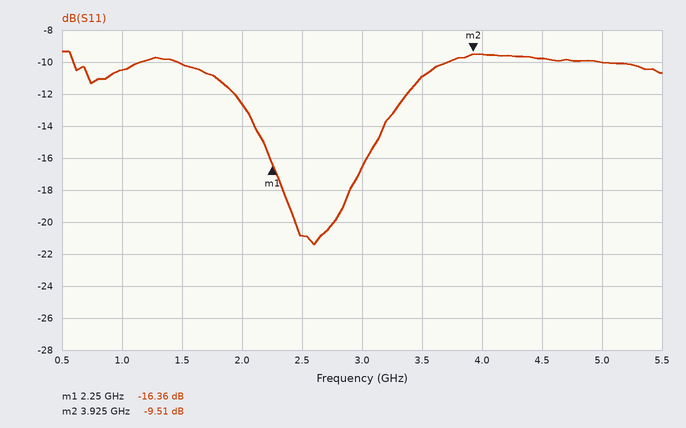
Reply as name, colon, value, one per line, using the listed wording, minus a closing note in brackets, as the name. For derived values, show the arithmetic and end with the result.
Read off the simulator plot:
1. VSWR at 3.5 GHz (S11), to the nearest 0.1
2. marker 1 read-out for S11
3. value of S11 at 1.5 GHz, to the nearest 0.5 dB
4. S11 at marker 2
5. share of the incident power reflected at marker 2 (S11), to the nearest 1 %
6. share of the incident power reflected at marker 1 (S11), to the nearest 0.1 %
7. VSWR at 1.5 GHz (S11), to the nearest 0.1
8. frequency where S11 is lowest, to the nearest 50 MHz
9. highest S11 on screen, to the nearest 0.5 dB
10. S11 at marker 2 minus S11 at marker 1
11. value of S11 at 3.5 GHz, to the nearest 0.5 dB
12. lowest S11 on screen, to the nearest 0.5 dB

VSWR at 3.5 GHz (S11), to the nearest 0.1: |Γ| = 10^(-11/20) = 0.2818; VSWR = (1 + 0.2818)/(1 − 0.2818) ≈ 1.8
marker 1 read-out for S11: -16.36 dB
value of S11 at 1.5 GHz, to the nearest 0.5 dB: -10.0 dB
S11 at marker 2: -9.51 dB
share of the incident power reflected at marker 2 (S11), to the nearest 1 %: 10^(-9.51/10) ≈ 11 %
share of the incident power reflected at marker 1 (S11), to the nearest 0.1 %: 10^(-16.36/10) ≈ 2.3 %
VSWR at 1.5 GHz (S11), to the nearest 0.1: |Γ| = 10^(-10/20) = 0.3162; VSWR = (1 + 0.3162)/(1 − 0.3162) ≈ 1.9
frequency where S11 is lowest, to the nearest 50 MHz: 2.60 GHz
highest S11 on screen, to the nearest 0.5 dB: -9.5 dB
S11 at marker 2 minus S11 at marker 1: -9.51 − (-16.36) = 6.85 dB
value of S11 at 3.5 GHz, to the nearest 0.5 dB: -11.0 dB
lowest S11 on screen, to the nearest 0.5 dB: -21.5 dB
